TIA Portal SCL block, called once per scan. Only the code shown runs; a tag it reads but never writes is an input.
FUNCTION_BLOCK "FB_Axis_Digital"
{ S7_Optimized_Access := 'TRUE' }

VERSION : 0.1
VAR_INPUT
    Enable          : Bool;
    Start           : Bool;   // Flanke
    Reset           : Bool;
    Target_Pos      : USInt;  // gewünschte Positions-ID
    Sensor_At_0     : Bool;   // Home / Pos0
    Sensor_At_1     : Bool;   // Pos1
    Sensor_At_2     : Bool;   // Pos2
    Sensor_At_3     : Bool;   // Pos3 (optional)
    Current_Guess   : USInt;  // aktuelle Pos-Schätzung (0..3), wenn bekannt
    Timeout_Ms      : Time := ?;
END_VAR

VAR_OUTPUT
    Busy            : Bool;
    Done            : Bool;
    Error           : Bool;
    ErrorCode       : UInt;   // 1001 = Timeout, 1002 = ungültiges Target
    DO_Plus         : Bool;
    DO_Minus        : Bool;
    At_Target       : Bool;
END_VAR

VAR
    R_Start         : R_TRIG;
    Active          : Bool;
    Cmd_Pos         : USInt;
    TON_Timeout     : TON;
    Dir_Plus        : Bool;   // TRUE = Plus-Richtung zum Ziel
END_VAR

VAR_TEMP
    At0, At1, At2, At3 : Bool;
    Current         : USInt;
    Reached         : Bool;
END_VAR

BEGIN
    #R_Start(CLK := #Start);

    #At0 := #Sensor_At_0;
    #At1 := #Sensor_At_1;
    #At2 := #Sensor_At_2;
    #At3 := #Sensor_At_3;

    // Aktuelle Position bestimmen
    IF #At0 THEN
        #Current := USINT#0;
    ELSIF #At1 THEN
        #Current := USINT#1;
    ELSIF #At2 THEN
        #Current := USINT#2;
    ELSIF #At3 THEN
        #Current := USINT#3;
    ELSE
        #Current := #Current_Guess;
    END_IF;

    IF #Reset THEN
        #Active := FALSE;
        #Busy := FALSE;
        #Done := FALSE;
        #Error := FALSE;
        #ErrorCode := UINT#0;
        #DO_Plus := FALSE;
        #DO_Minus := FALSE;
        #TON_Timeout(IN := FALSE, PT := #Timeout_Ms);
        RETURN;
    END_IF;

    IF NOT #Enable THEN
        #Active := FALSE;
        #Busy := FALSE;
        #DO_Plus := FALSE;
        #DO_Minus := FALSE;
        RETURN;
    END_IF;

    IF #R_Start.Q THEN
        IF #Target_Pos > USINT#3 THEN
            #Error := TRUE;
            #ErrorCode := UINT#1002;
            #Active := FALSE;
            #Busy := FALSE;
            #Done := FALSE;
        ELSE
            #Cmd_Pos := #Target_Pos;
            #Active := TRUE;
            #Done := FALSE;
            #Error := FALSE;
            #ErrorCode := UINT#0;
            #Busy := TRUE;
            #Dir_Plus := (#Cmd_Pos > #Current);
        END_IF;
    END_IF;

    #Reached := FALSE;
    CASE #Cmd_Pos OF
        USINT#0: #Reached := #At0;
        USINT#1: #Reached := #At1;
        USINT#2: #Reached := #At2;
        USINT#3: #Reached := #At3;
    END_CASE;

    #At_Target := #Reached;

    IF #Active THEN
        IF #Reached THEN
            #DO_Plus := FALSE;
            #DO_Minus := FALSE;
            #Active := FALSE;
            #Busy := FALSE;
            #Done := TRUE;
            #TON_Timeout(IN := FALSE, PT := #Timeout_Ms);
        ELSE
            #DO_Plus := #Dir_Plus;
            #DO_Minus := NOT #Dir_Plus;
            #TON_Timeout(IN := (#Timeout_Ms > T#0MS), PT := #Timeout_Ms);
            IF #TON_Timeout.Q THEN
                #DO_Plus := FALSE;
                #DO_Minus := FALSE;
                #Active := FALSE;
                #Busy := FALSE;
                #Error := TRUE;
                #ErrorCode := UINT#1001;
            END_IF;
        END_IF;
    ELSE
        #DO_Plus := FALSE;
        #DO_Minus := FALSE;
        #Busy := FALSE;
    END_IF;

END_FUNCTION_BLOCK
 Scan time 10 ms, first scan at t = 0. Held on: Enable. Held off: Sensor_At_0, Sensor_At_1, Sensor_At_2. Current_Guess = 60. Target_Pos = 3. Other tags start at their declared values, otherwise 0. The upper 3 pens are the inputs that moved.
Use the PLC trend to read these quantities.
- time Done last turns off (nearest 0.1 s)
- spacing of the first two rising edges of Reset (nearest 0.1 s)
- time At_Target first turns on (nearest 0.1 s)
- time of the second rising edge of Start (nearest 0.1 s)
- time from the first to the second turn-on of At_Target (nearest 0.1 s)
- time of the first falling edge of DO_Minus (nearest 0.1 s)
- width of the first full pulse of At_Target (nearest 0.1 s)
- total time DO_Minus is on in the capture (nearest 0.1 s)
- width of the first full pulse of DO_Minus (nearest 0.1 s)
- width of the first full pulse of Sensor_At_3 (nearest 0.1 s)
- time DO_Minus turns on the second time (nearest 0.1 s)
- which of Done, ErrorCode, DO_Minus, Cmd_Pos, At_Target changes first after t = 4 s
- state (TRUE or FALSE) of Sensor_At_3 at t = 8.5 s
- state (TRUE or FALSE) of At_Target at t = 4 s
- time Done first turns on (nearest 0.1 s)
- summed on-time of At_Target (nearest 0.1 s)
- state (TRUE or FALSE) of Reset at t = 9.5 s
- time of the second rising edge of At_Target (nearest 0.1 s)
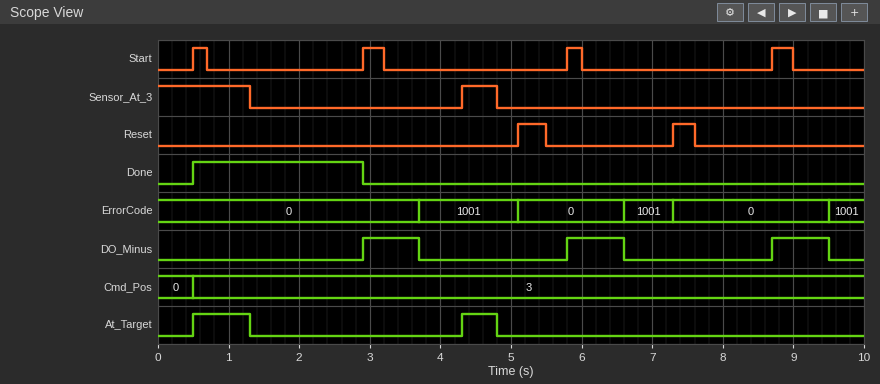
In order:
2.9 s
2.2 s
0.5 s
2.9 s
3.8 s
3.7 s
0.8 s
2.4 s
0.8 s
0.5 s
5.8 s
At_Target
FALSE
FALSE
0.5 s
1.3 s
FALSE
4.3 s
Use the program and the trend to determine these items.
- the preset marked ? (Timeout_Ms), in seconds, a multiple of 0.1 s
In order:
0.8 s
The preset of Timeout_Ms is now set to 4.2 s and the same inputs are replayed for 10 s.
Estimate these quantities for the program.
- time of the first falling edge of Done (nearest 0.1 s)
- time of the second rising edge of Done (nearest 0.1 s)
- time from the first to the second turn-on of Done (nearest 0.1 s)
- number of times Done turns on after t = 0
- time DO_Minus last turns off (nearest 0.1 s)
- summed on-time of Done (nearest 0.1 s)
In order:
2.9 s
4.3 s
3.8 s
2
7.3 s
3.2 s
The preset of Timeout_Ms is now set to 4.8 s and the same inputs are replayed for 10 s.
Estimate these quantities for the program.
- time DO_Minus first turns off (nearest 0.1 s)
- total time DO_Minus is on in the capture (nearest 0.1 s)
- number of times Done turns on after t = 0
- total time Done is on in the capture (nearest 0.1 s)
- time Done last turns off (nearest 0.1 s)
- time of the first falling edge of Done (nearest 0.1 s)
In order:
4.3 s
4.2 s
2
3.2 s
5.1 s
2.9 s
